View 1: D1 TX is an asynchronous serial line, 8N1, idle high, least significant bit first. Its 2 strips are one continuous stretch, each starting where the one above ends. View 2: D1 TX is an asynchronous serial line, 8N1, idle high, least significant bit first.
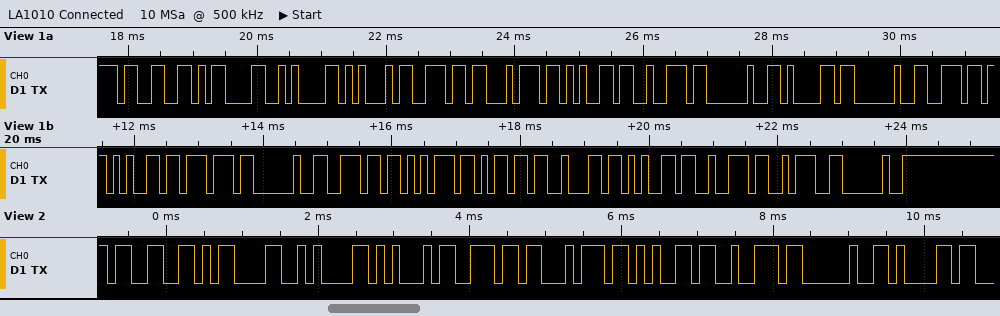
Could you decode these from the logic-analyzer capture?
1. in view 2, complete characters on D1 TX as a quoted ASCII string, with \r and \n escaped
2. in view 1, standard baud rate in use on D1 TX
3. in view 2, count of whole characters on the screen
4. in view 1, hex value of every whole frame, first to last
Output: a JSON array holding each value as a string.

["\"3\\r\\nEnter a\"", "9600 baud", "10", "33 0D 0A 45 6E 74 65 72 20 61 20 6E 65 77 20 6E 75 6D 62 65 72 3A 20"]
